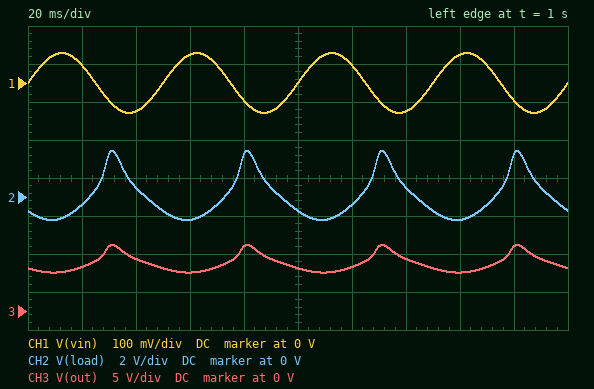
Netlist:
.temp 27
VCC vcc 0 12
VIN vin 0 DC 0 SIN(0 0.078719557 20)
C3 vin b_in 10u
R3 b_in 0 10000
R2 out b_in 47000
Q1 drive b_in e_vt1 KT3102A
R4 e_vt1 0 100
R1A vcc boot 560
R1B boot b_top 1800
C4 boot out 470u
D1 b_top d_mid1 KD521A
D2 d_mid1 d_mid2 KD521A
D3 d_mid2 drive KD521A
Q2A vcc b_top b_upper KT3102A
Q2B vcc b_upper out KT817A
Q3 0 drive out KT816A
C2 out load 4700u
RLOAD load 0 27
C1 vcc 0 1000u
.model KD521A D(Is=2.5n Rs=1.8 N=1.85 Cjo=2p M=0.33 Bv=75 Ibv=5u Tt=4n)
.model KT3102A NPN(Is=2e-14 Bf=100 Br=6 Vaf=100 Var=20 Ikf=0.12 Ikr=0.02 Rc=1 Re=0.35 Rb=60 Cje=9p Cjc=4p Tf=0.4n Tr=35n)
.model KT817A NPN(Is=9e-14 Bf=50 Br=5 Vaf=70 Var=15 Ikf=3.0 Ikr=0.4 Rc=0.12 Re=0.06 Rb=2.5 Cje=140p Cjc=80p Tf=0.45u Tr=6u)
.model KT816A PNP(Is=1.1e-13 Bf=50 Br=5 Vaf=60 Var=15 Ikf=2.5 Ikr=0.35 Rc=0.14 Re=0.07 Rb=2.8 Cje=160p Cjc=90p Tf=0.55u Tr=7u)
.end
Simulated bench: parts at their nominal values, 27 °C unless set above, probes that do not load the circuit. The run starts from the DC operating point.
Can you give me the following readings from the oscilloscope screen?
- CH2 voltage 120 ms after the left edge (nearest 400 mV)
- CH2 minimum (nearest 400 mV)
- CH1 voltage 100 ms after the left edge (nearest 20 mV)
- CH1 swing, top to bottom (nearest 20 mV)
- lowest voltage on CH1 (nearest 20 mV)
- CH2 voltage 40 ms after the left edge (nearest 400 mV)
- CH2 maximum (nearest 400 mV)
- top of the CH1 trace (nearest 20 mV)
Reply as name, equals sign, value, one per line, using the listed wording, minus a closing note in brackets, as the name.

CH2 voltage 120 ms after the left edge = -400 mV
CH2 minimum = -1.2 V
CH1 voltage 100 ms after the left edge = 0 V
CH1 swing, top to bottom = 160 mV
lowest voltage on CH1 = -80 mV
CH2 voltage 40 ms after the left edge = 400 mV
CH2 maximum = 2.4 V
top of the CH1 trace = 80 mV
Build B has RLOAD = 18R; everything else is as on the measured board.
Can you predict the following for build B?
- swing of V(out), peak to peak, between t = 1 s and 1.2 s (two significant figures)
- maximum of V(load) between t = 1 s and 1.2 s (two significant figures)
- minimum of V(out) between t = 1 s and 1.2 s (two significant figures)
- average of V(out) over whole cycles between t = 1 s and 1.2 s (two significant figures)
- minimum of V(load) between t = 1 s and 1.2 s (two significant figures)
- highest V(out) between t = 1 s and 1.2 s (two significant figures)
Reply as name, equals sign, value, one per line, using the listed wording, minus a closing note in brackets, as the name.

swing of V(out), peak to peak, between t = 1 s and 1.2 s = 2.9 V
maximum of V(load) between t = 1 s and 1.2 s = 2.0 V
minimum of V(out) between t = 1 s and 1.2 s = 5.4 V
average of V(out) over whole cycles between t = 1 s and 1.2 s = 6.3 V
minimum of V(load) between t = 1 s and 1.2 s = -890 mV
highest V(out) between t = 1 s and 1.2 s = 8.3 V
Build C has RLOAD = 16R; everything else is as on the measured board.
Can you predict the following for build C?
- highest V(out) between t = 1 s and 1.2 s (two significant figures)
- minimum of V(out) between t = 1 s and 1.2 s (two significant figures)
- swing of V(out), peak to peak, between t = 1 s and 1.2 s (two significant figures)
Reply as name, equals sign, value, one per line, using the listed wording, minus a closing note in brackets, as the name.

highest V(out) between t = 1 s and 1.2 s = 8.1 V
minimum of V(out) between t = 1 s and 1.2 s = 5.5 V
swing of V(out), peak to peak, between t = 1 s and 1.2 s = 2.6 V
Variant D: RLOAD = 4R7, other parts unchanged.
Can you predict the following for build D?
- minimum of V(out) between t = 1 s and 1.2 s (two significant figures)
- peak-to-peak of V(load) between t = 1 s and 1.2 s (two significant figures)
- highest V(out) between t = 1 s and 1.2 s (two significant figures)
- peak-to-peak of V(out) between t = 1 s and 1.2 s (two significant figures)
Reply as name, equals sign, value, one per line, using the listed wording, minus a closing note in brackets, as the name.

minimum of V(out) between t = 1 s and 1.2 s = 6.0 V
peak-to-peak of V(load) between t = 1 s and 1.2 s = 970 mV
highest V(out) between t = 1 s and 1.2 s = 7.0 V
peak-to-peak of V(out) between t = 1 s and 1.2 s = 990 mV
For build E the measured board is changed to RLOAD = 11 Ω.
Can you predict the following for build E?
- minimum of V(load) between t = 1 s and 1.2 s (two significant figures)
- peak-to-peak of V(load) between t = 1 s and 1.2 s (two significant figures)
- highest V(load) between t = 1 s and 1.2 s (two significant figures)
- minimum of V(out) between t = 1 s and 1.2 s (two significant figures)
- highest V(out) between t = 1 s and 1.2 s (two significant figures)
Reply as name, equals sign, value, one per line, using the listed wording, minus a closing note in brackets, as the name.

minimum of V(load) between t = 1 s and 1.2 s = -580 mV
peak-to-peak of V(load) between t = 1 s and 1.2 s = 2.0 V
highest V(load) between t = 1 s and 1.2 s = 1.4 V
minimum of V(out) between t = 1 s and 1.2 s = 5.7 V
highest V(out) between t = 1 s and 1.2 s = 7.7 V
